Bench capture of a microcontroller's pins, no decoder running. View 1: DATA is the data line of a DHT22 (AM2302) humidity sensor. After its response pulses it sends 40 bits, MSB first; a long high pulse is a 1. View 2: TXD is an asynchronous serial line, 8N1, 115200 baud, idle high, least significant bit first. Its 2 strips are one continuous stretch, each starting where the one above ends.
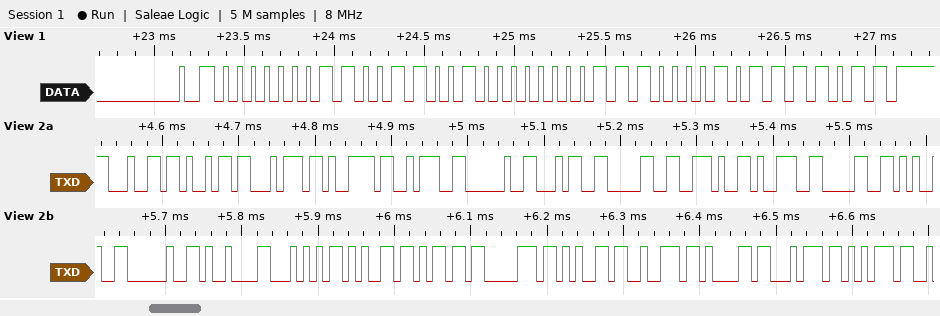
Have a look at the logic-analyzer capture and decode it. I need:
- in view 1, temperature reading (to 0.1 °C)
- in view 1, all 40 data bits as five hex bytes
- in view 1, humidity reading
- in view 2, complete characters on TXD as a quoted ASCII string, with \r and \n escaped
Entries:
22.5 °C
01 99 00 E1 7B
40.9 %
"dity: 40.90% \tTemperatu"
